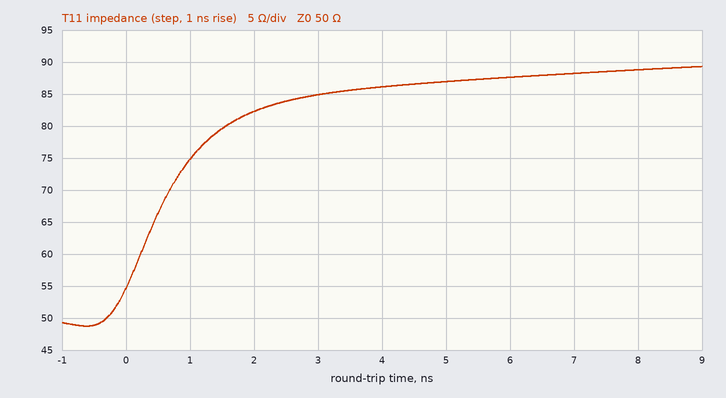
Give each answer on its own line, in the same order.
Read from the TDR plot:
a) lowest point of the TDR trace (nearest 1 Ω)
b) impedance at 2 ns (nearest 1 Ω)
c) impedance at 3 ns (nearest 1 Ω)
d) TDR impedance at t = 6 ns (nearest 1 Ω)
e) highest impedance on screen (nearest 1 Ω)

49 Ω
82 Ω
85 Ω
88 Ω
89 Ω
